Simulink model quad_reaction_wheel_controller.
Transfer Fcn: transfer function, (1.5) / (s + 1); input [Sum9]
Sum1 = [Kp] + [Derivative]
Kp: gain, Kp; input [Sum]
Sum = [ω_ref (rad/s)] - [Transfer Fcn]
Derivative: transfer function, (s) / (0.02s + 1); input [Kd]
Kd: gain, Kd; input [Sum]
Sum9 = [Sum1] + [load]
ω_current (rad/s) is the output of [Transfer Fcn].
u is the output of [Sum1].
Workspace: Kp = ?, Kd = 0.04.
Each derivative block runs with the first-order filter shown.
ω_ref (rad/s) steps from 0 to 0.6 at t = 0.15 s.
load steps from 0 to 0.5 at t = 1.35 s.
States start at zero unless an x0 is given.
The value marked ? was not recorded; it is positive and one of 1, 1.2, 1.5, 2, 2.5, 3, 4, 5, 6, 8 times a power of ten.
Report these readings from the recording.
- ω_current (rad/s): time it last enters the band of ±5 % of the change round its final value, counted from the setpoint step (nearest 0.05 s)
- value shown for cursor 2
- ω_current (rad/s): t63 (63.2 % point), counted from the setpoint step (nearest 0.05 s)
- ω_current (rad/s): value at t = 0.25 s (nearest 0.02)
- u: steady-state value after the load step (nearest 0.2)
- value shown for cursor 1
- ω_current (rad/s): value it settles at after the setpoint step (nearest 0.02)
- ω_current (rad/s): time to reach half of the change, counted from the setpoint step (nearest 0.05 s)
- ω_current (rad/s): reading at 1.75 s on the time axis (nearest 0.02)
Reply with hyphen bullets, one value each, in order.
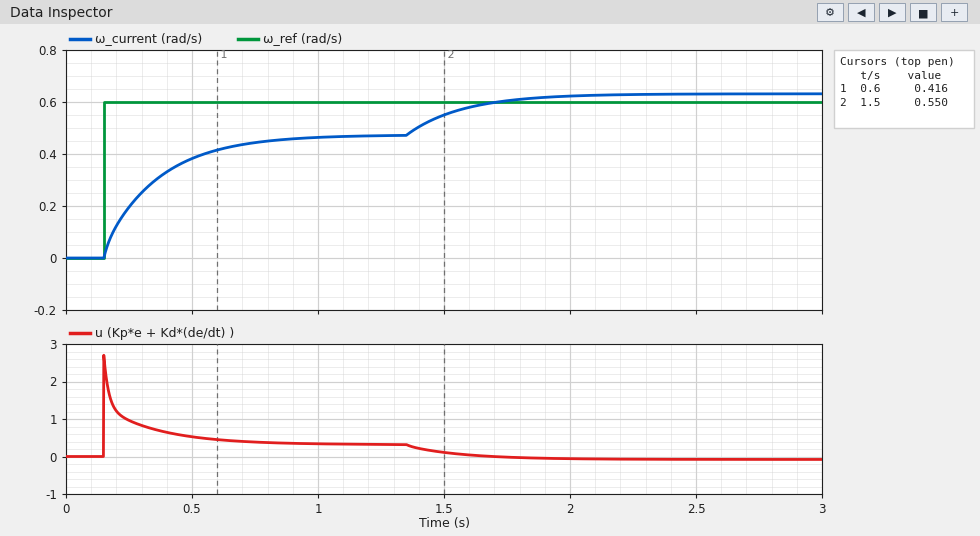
- 0.65 s
- 0.550
- 0.20 s
- 0.20
- 0.0
- 0.416
- 0.48
- 0.15 s
- 0.60
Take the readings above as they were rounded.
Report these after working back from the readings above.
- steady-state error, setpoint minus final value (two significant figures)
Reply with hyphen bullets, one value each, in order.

- 0.12
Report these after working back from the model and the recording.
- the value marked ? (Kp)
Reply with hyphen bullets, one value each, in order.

- 2.5
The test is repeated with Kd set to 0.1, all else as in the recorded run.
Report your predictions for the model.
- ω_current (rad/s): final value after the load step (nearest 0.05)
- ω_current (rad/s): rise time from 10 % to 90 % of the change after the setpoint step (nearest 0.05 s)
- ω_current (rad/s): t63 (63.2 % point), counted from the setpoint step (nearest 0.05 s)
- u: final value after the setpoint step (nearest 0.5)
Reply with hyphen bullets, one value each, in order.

- 0.65
- 0.50 s
- 0.20 s
- 0.5
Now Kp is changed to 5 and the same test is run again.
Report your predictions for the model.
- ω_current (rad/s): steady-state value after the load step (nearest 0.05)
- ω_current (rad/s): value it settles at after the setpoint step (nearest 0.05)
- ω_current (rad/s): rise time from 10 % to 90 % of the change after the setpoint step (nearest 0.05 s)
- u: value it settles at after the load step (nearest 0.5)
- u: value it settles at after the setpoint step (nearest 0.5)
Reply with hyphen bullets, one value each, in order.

- 0.60
- 0.55
- 0.25 s
- 0.0
- 0.5
